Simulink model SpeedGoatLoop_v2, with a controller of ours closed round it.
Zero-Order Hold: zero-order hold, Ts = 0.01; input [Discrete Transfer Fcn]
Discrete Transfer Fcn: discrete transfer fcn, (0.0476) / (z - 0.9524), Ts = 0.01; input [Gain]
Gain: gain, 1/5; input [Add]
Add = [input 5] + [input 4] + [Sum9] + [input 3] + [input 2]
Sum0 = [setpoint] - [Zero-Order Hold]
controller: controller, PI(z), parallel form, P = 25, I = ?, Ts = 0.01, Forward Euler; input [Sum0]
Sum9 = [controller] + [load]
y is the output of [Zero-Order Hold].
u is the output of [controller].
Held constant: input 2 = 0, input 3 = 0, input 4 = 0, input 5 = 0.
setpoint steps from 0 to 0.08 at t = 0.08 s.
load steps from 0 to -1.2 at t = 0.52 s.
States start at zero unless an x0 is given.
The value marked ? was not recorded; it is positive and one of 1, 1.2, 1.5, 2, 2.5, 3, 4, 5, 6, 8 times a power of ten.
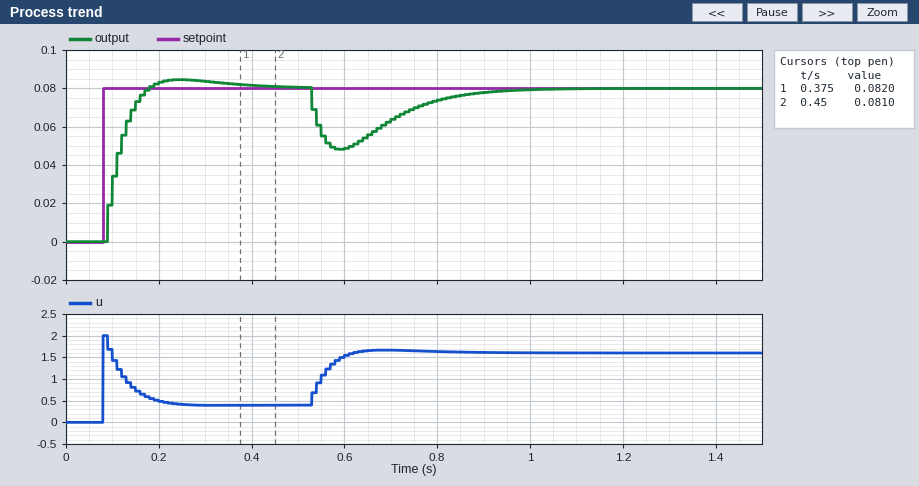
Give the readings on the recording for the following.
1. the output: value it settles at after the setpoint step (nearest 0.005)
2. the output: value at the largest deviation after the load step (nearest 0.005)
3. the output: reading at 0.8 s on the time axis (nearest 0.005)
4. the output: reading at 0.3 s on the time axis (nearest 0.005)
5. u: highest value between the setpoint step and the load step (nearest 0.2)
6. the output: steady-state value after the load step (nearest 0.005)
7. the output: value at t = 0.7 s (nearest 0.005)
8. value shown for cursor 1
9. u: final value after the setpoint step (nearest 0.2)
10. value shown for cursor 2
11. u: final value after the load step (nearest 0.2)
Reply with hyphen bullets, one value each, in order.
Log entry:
- 0.080
- 0.050
- 0.075
- 0.085
- 2.0
- 0.080
- 0.065
- 0.0820
- 0.4
- 0.0810
- 1.6
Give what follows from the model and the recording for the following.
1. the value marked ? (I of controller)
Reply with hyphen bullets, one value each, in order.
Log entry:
- 200
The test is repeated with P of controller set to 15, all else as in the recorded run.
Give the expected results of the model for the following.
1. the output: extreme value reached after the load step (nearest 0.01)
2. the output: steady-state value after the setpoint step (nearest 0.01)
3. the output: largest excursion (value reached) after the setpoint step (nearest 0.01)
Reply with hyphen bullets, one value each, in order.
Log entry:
- 0.04
- 0.08
- 0.09
